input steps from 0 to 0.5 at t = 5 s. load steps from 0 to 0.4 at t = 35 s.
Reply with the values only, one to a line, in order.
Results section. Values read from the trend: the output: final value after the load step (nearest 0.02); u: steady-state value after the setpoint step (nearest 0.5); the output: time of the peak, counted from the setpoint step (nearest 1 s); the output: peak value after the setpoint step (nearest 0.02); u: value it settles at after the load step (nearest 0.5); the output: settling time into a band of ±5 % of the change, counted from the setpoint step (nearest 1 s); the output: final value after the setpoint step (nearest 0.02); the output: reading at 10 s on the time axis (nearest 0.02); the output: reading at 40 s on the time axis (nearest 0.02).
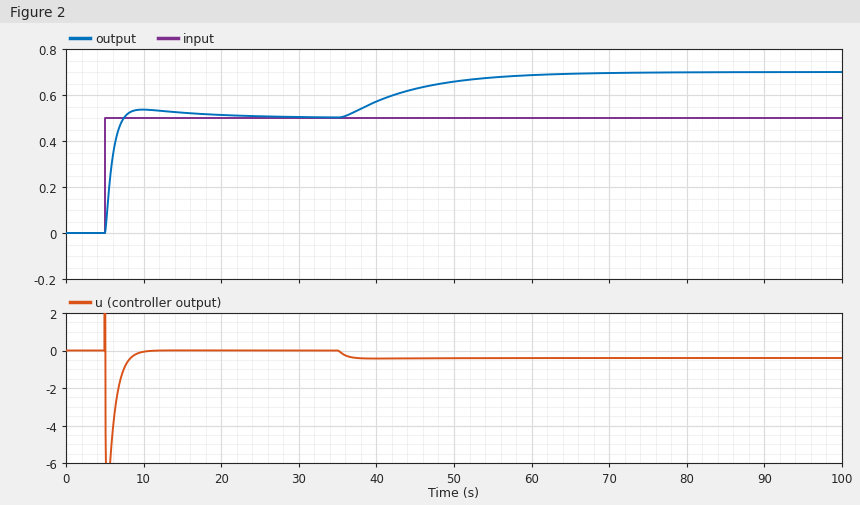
0.70
0.0
5 s
0.54
-0.5
9 s
0.50
0.54
0.58
